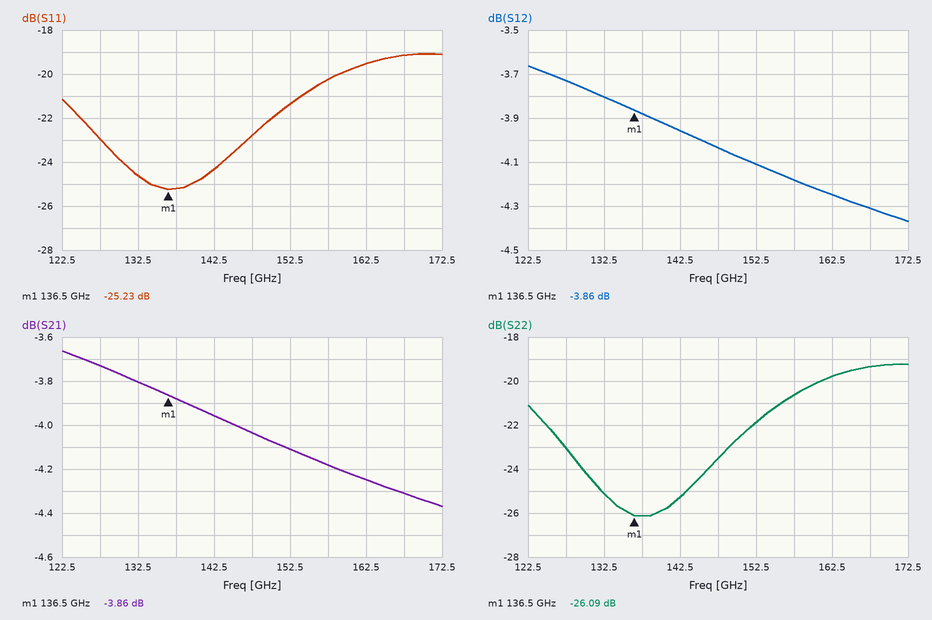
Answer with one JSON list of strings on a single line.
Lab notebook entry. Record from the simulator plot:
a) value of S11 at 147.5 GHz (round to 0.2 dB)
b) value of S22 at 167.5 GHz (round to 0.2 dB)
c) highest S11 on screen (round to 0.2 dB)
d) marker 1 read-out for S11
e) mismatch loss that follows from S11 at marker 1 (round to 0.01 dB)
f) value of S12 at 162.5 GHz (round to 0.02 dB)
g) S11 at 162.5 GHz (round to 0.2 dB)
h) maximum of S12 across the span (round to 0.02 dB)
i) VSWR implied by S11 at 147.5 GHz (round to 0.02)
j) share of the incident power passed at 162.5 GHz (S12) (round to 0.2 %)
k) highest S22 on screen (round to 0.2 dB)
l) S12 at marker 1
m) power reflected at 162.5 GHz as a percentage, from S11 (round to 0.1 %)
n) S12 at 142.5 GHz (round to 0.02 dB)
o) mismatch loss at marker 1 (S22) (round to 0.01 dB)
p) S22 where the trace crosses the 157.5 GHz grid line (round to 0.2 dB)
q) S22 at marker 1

["-22.8 dB", "-19.4 dB", "-19.0 dB", "-25.23 dB", "0.01 dB", "-4.24 dB", "-19.6 dB", "-3.66 dB", "1.16", "37.6 %", "-19.2 dB", "-3.86 dB", "1.1 %", "-3.96 dB", "0.01 dB", "-20.6 dB", "-26.09 dB"]
